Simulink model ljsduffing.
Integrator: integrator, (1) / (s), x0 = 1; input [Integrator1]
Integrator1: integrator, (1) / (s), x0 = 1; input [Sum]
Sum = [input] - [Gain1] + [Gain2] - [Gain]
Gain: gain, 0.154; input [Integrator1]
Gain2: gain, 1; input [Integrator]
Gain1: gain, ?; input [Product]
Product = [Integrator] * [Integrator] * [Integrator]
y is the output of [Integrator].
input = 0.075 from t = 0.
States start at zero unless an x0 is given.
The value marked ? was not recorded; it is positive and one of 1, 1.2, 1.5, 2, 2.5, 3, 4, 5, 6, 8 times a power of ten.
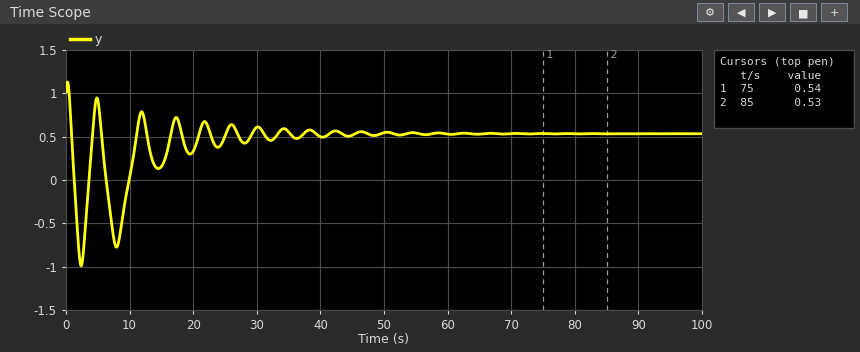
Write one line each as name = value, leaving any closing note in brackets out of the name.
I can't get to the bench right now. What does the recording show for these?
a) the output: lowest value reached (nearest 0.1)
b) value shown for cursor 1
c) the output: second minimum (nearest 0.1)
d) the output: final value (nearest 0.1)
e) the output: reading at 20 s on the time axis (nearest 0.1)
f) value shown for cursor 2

the output: lowest value reached = -1.0
value shown for cursor 1 = 0.54
the output: second minimum = -0.8
the output: final value = 0.5
the output: reading at 20 s on the time axis = 0.3
value shown for cursor 2 = 0.53
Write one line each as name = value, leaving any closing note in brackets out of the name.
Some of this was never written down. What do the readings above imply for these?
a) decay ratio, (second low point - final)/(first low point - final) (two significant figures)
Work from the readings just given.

decay ratio, (second low point - final)/(first low point - final) = 0.87
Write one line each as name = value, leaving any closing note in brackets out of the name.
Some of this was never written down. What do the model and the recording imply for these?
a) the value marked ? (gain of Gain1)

the value marked ? = 4
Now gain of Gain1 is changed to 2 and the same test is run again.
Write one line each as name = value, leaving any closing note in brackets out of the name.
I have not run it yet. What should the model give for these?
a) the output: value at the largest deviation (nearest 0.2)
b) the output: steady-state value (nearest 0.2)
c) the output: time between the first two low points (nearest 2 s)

the output: value at the largest deviation = -1.0
the output: steady-state value = 0.8
the output: time between the first two low points = 8 s
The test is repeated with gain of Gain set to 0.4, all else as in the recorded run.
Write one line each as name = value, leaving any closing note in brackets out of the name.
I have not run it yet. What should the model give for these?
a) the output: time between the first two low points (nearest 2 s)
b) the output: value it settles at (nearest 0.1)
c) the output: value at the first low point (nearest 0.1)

the output: time between the first two low points = 6 s
the output: value it settles at = 0.5
the output: value at the first low point = -0.8
